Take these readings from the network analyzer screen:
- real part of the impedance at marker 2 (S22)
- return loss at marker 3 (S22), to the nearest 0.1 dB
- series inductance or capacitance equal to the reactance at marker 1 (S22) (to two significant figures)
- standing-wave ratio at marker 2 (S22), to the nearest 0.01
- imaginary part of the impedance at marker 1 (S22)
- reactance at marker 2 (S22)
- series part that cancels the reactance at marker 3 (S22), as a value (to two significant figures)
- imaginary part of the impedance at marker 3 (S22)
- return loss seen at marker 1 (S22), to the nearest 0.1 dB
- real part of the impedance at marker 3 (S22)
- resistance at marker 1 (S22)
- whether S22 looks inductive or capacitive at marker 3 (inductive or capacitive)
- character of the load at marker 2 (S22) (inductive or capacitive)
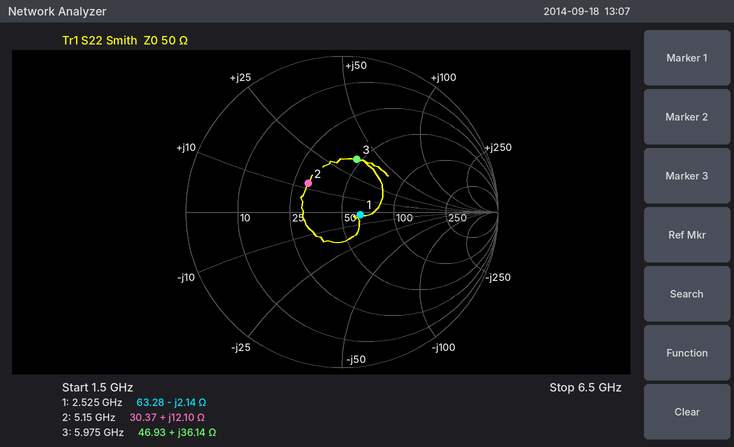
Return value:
30.37 Ω
9.1 dB
29 pF
1.79
-2.14 Ω
+12.10 Ω
740 fF
+36.14 Ω
18.5 dB
46.93 Ω
63.28 Ω
inductive
inductive
